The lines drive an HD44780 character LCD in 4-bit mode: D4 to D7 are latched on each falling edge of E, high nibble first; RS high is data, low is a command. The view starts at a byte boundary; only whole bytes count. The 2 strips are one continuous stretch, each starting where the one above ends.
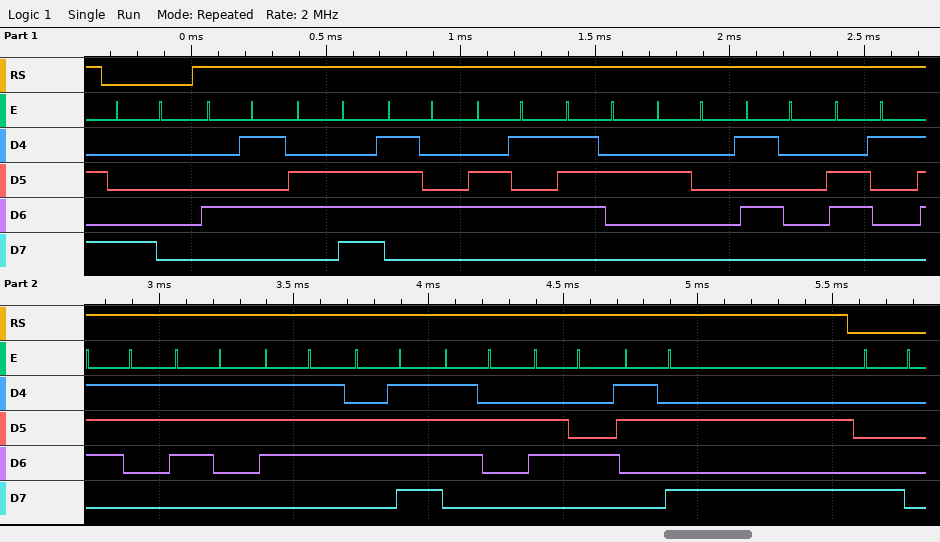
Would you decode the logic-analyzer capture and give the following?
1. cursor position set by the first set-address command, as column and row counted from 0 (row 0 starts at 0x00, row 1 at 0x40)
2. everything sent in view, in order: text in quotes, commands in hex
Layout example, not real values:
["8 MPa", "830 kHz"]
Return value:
["column 0, row 0", "0x80 \"Enter Password:\" 0x80"]
